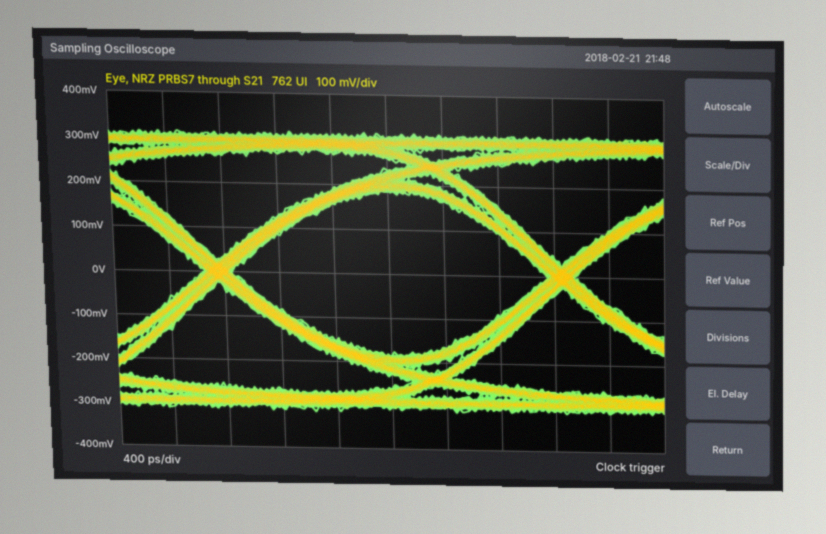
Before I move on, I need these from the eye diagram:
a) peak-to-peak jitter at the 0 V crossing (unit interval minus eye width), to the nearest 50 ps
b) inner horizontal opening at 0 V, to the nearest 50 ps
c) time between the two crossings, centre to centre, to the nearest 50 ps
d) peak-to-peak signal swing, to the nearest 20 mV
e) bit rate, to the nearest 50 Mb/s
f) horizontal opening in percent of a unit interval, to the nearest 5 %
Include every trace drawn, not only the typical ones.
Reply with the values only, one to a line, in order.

200 ps
2.30 ns
2.50 ns
640 mV
400 Mb/s
90 %
